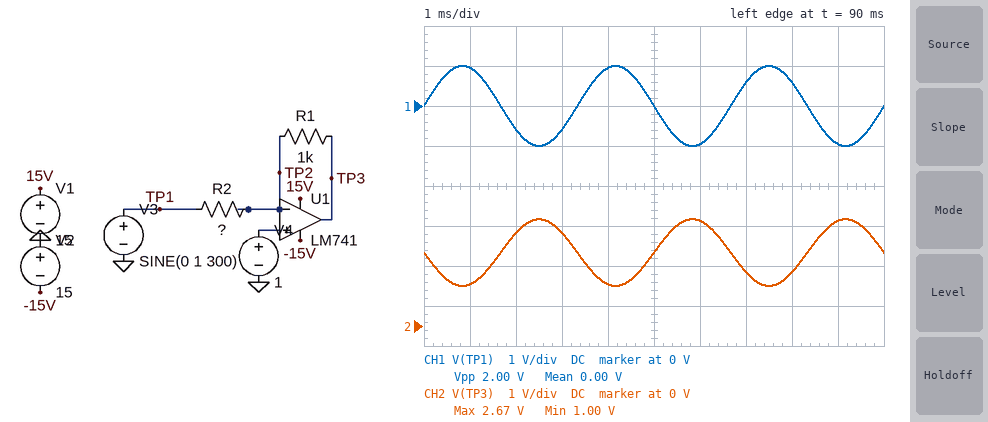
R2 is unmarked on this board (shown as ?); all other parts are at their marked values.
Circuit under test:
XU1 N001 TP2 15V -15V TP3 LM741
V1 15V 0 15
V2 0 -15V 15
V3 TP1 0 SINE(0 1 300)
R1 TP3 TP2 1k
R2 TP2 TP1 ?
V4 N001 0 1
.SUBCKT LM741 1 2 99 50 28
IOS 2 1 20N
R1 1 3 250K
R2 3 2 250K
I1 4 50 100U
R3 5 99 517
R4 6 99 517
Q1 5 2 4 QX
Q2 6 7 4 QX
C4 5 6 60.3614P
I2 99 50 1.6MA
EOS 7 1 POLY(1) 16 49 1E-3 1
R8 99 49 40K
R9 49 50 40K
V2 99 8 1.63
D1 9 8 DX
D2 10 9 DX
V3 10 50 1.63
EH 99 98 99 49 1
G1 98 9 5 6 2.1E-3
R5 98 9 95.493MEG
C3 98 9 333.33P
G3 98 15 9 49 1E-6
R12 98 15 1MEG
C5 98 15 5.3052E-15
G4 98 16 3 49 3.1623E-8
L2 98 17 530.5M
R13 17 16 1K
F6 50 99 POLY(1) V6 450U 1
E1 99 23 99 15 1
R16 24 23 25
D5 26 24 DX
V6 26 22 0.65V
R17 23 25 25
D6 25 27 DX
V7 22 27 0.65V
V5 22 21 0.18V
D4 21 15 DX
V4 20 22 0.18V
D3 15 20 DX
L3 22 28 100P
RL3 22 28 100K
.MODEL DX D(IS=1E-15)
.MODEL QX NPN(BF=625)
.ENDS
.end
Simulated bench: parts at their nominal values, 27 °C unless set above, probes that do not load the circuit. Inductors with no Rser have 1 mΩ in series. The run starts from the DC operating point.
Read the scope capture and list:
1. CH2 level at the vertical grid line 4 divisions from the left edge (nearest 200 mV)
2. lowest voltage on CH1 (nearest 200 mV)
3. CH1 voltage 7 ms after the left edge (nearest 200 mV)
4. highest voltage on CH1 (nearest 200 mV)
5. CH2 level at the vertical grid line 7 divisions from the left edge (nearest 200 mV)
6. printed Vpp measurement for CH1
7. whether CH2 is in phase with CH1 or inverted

1.0 V
-1.0 V
600 mV
1.0 V
1.4 V
2.00 V
inverted
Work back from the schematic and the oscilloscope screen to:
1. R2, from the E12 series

1.2 kΩ
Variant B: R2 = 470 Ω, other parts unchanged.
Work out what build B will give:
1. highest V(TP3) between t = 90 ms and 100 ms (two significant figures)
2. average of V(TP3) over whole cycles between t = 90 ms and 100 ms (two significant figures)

5.3 V
3.1 V
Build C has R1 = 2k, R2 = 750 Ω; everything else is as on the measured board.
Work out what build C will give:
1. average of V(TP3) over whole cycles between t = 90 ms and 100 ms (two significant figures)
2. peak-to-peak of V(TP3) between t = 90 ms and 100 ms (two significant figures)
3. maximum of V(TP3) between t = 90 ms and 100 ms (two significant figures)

3.7 V
5.3 V
6.3 V
